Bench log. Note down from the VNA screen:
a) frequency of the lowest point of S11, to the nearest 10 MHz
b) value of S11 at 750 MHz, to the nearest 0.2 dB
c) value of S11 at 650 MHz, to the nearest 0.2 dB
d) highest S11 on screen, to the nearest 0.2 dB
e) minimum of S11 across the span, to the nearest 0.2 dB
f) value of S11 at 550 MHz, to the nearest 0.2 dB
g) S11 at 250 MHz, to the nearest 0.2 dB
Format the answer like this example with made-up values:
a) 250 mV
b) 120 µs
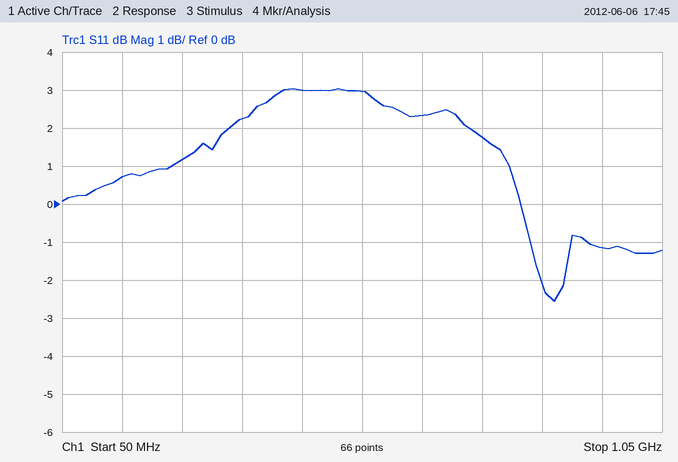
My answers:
a) 870 MHz
b) 1.8 dB
c) 2.4 dB
d) 3.0 dB
e) -2.6 dB
f) 3.0 dB
g) 1.2 dB
